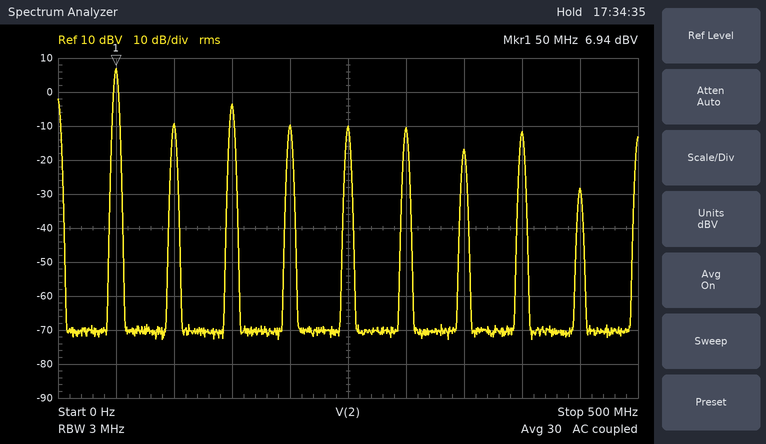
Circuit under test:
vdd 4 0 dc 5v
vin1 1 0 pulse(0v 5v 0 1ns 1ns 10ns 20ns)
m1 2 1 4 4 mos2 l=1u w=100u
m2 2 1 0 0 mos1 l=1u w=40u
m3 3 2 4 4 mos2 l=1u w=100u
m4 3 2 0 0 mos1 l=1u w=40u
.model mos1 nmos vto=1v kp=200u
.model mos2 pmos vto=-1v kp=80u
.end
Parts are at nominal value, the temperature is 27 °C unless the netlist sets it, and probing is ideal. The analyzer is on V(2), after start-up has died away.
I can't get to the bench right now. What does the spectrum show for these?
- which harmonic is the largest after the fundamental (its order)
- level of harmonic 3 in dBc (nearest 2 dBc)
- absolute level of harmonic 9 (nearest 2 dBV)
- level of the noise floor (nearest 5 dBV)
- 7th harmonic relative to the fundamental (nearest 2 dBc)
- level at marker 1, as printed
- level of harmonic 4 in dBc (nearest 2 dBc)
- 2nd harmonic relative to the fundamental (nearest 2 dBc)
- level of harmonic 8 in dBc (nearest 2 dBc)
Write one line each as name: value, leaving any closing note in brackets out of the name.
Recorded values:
which harmonic is the largest after the fundamental: 3
level of harmonic 3 in dBc: -10 dBc
absolute level of harmonic 9: -28 dBV
level of the noise floor: -70 dBV
7th harmonic relative to the fundamental: -24 dBc
level at marker 1, as printed: 6.94 dBV
level of harmonic 4 in dBc: -16 dBc
2nd harmonic relative to the fundamental: -16 dBc
level of harmonic 8 in dBc: -18 dBc
